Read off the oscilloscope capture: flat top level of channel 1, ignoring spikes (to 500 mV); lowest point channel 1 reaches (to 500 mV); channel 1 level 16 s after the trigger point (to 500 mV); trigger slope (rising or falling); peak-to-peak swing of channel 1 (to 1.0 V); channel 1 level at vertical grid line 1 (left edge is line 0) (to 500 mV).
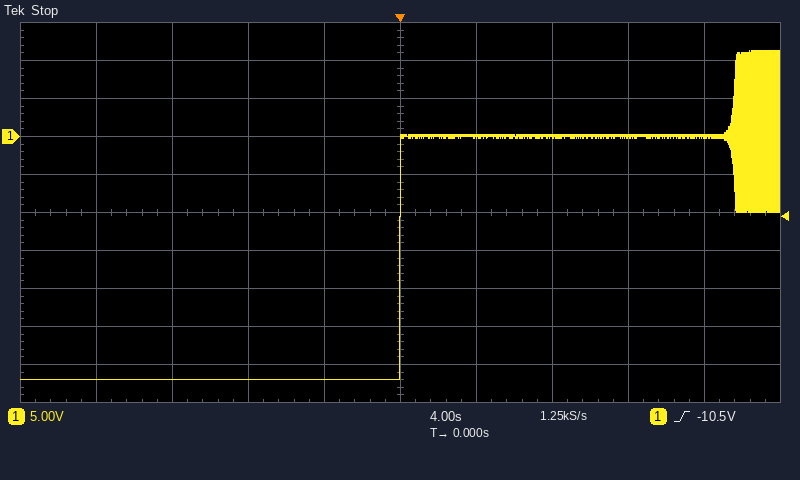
0.0 V
-32.0 V
0.0 V
rising
43.0 V
-32.0 V
